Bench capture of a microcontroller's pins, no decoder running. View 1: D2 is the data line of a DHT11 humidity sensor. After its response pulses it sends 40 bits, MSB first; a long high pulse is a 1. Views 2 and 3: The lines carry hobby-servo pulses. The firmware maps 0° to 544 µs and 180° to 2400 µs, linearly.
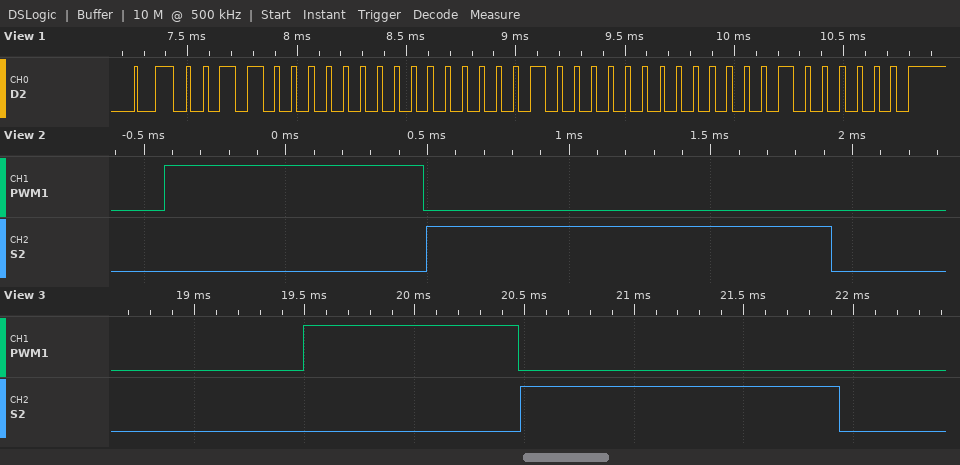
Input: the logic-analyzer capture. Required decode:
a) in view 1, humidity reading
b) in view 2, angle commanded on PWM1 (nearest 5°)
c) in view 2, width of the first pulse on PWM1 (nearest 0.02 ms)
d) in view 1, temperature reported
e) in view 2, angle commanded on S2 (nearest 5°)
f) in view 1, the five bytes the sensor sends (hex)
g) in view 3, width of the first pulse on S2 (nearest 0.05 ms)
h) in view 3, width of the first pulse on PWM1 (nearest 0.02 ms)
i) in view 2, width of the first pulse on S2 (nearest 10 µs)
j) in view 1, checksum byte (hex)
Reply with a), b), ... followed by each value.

a) 48 %
b) 35°
c) 0.92 ms
d) 16.0 °C
e) 85°
f) 30 00 10 00 40
g) 1.45 ms
h) 0.98 ms
i) 1430 µs
j) 0x40
